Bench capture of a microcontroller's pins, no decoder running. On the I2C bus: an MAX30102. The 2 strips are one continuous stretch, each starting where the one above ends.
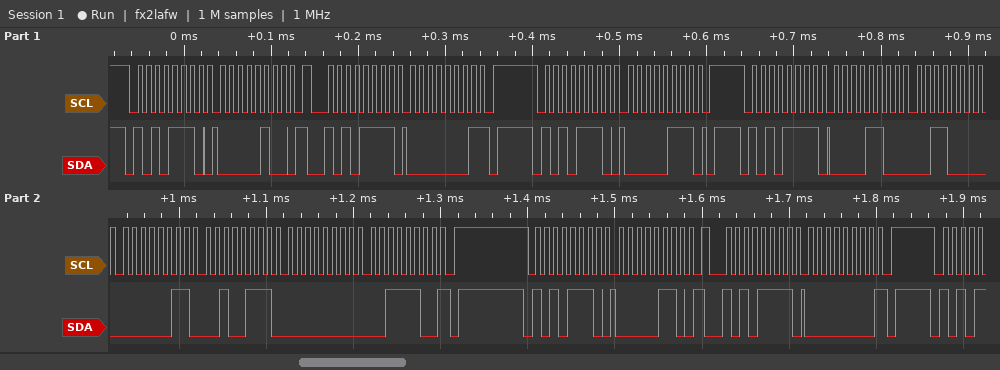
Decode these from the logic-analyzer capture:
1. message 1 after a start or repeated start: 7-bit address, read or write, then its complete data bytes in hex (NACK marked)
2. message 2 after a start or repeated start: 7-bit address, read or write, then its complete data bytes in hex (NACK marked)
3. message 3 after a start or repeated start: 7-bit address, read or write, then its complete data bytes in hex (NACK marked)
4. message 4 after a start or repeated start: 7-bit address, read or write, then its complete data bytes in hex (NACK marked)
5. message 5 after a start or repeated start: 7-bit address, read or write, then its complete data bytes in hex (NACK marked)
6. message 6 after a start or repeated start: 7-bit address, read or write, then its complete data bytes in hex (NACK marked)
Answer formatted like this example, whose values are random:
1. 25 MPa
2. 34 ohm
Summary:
1. 0x57 write: 04
2. 0x57 read: 01 NACK
3. 0x57 write: 07
4. 0x57 read: 0C 30 03 27 00 3C NACK
5. 0x57 write: 06
6. 0x57 read: 00 NACK
